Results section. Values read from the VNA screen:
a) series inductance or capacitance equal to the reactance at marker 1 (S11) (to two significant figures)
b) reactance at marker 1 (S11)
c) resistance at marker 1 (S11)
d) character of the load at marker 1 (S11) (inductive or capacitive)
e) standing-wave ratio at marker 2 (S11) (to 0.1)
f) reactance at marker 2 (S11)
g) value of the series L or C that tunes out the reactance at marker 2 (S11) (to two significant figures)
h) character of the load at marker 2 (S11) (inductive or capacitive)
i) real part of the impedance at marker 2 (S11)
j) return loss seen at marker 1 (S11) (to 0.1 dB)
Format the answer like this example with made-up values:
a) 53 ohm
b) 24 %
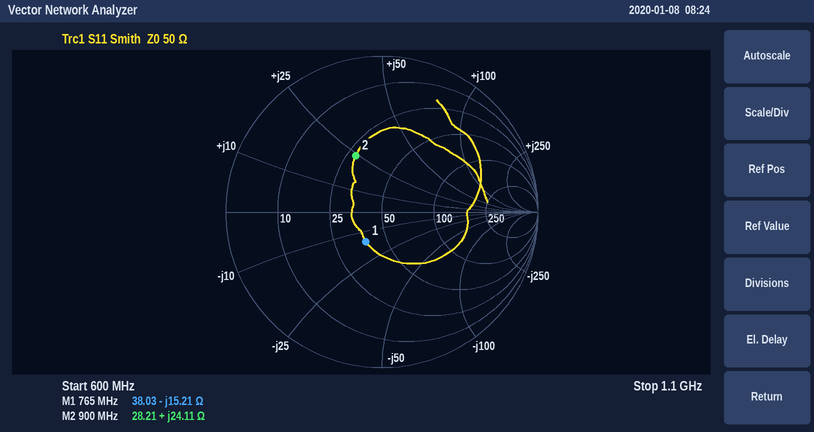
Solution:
a) 14 pF
b) -15.21 Ω
c) 38.03 Ω
d) capacitive
e) 2.3
f) +24.11 Ω
g) 7.3 pF
h) inductive
i) 28.21 Ω
j) 13.3 dB
